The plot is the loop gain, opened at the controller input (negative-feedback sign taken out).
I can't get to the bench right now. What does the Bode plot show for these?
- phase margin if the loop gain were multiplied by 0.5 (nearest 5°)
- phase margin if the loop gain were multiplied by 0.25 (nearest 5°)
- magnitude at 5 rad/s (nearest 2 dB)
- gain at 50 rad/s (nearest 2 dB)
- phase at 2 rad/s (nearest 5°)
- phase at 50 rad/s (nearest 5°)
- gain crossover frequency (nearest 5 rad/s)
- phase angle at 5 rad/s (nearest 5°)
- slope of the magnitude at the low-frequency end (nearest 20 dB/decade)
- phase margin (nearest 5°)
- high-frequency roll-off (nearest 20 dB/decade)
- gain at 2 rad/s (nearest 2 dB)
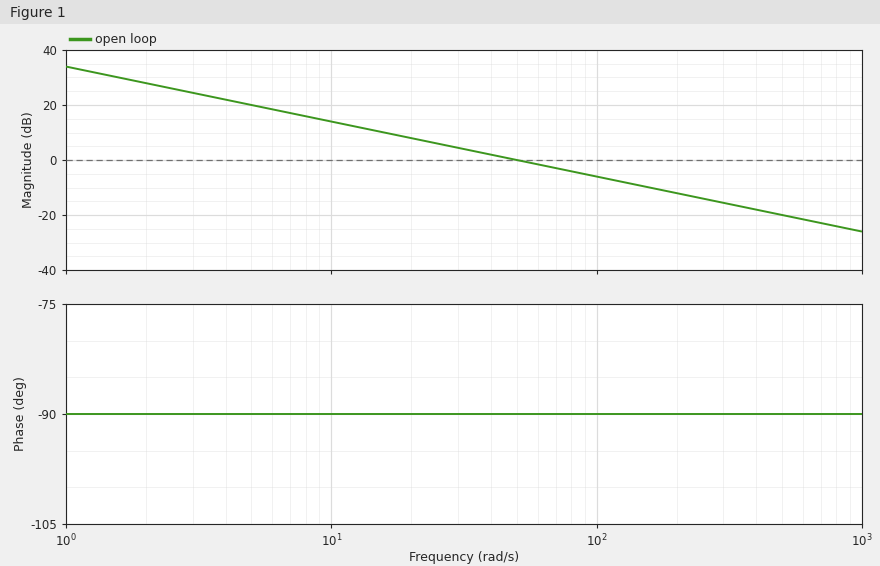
90°
90°
20 dB
0 dB
-90°
-90°
50 rad/s
-90°
-20 dB/decade
90°
-20 dB/decade
28 dB
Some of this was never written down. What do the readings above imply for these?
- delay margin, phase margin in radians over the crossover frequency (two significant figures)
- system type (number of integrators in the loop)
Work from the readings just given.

0.031 s
1
